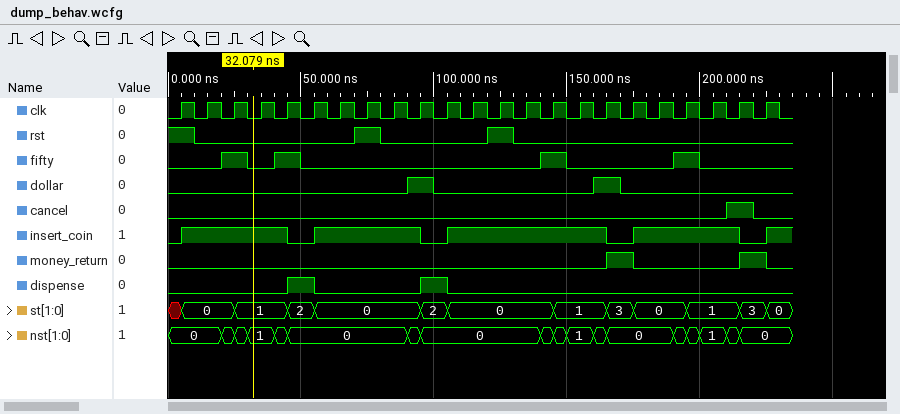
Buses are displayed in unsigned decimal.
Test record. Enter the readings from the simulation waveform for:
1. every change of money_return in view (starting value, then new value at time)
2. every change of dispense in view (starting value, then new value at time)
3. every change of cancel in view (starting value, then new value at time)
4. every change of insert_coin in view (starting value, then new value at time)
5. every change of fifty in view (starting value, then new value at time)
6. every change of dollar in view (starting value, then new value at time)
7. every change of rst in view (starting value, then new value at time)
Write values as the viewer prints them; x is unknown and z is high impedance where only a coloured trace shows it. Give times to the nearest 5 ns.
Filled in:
0, 1 at 165 ns, 0 at 175 ns, 1 at 215 ns, 0 at 225 ns
0, 1 at 45 ns, 0 at 55 ns, 1 at 95 ns, 0 at 105 ns
0, 1 at 210 ns, 0 at 220 ns
0, 1 at 5 ns, 0 at 45 ns, 1 at 55 ns, 0 at 95 ns, 1 at 105 ns, 0 at 165 ns, 1 at 175 ns, 0 at 215 ns, 1 at 225 ns
0, 1 at 20 ns, 0 at 30 ns, 1 at 40 ns, 0 at 50 ns, 1 at 140 ns, 0 at 150 ns, 1 at 190 ns, 0 at 200 ns
0, 1 at 90 ns, 0 at 100 ns, 1 at 160 ns, 0 at 170 ns
1, 0 at 10 ns, 1 at 70 ns, 0 at 80 ns, 1 at 120 ns, 0 at 130 ns
